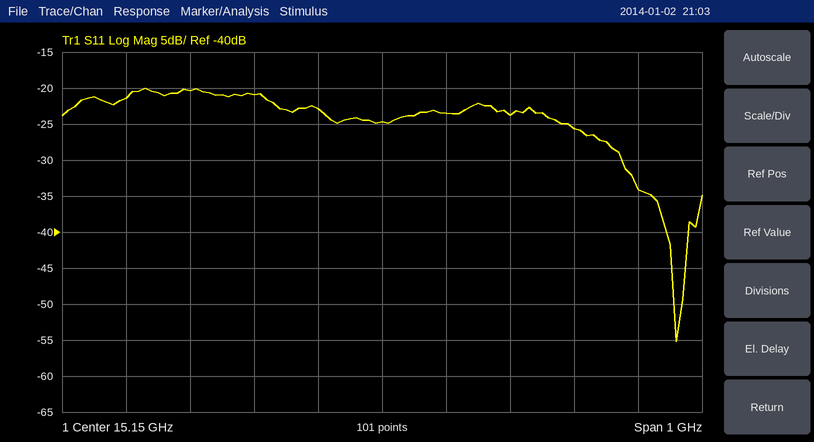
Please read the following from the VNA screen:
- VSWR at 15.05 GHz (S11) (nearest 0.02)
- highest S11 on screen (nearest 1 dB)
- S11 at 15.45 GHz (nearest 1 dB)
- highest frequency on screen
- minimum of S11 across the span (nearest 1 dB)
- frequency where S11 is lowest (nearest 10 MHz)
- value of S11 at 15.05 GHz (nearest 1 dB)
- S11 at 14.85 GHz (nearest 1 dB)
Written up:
1.16
-20 dB
-26 dB
15.65 GHz
-55 dB
15.61 GHz
-23 dB
-20 dB
